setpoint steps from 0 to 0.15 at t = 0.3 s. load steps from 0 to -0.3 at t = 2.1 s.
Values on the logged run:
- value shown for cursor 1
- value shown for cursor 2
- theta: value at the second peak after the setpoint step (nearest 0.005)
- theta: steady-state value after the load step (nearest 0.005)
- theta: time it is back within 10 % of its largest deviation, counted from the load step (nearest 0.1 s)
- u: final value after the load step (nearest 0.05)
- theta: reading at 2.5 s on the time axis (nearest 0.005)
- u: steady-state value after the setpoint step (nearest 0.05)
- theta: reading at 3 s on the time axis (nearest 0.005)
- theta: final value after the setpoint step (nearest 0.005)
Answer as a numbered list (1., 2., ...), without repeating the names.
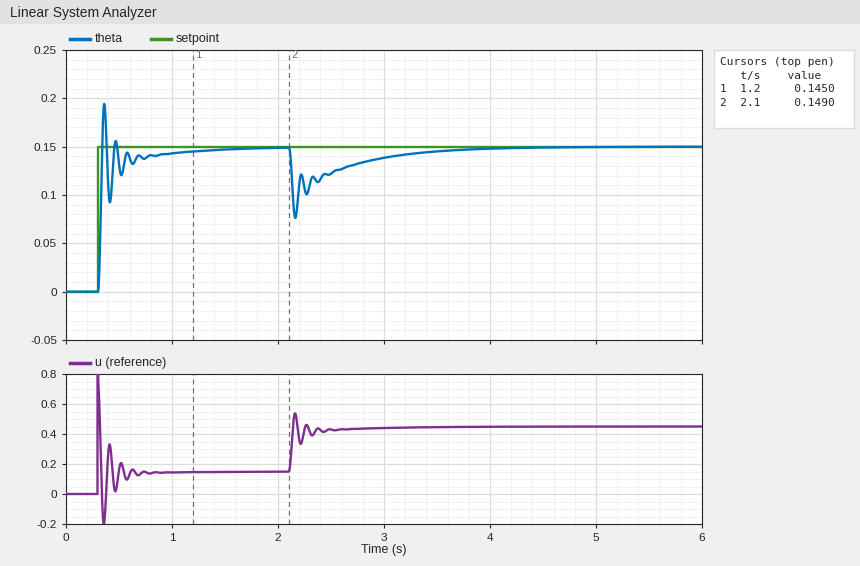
1. 0.1450
2. 0.1490
3. 0.155
4. 0.150
5. 1.2 s
6. 0.45
7. 0.120
8. 0.15
9. 0.140
10. 0.150
